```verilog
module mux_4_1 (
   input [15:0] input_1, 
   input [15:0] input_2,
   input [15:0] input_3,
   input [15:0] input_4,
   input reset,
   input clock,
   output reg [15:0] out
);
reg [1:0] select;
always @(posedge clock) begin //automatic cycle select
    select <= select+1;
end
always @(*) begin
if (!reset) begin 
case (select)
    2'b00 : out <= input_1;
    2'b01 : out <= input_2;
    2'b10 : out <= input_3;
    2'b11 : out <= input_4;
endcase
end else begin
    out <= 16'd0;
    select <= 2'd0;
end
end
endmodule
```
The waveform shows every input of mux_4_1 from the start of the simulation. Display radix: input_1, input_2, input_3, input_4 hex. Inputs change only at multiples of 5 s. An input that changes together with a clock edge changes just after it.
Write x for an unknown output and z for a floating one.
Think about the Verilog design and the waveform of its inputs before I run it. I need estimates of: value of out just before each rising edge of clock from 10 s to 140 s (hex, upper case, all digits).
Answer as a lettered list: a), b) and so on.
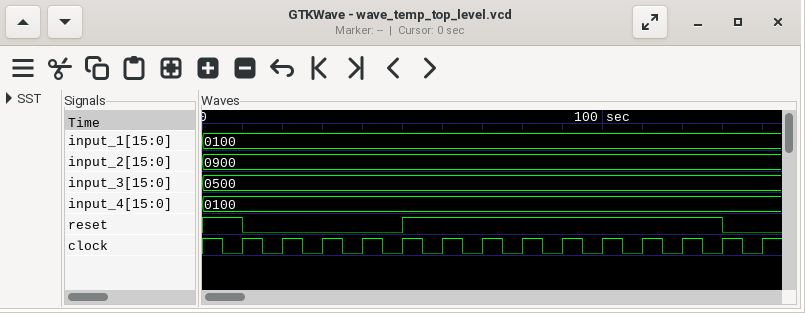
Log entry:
a) 0000, 0100, 0900, 0500, 0100, 0000, 0000, 0000, 0000, 0000, 0000, 0000, 0000, 0100
